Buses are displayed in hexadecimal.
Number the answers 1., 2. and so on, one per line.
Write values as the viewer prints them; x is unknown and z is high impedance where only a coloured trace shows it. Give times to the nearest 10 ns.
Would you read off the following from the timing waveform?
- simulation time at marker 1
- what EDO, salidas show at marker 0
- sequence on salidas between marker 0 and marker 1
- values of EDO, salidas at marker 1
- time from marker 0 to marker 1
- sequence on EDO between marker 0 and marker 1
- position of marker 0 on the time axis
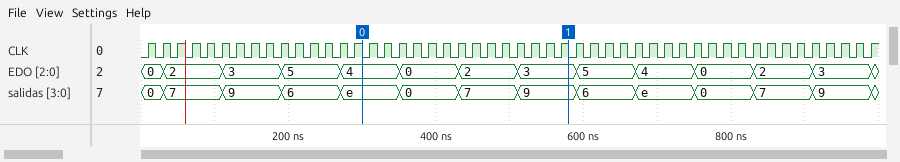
1. 580 ns
2. EDO=4, salidas=e
3. e, 0, 7, 9
4. EDO=3, salidas=9
5. 280 ns
6. 4, 0, 2, 3
7. 300 ns
